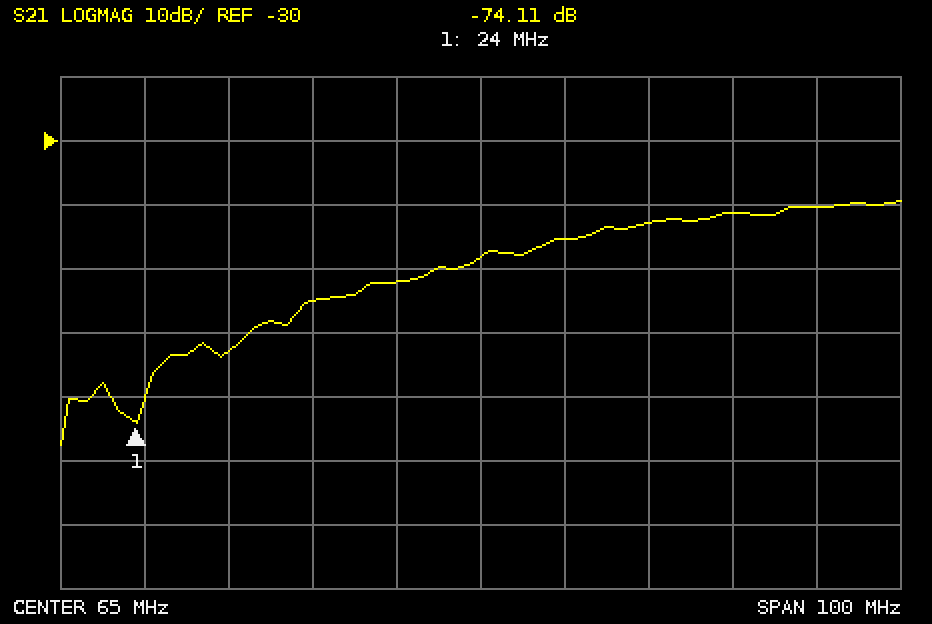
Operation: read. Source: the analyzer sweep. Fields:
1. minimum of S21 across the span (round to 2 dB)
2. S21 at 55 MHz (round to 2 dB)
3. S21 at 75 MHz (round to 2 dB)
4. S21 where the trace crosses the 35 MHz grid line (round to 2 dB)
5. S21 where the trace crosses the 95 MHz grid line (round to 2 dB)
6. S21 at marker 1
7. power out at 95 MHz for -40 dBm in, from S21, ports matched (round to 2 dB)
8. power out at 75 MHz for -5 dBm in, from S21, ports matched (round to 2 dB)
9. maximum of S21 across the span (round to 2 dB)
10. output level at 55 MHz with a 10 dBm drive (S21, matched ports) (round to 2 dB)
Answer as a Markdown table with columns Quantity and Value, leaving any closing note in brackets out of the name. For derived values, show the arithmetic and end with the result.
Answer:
| Quantity | Value |
|---|---|
| minimum of S21 across the span | -78 dB |
| S21 at 55 MHz | -52 dB |
| S21 at 75 MHz | -46 dB |
| S21 where the trace crosses the 35 MHz grid line | -62 dB |
| S21 where the trace crosses the 95 MHz grid line | -42 dB |
| S21 at marker 1 | -74.11 dB |
| power out at 95 MHz for -40 dBm in, from S21, ports matched | -40 dBm + (-42 dB) = -82 dBm |
| power out at 75 MHz for -5 dBm in, from S21, ports matched | -5 dBm + (-46 dB) = -50 dBm |
| maximum of S21 across the span | -40 dB |
| output level at 55 MHz with a 10 dBm drive (S21, matched ports) | 10 dBm + (-52 dB) = -42 dBm |
